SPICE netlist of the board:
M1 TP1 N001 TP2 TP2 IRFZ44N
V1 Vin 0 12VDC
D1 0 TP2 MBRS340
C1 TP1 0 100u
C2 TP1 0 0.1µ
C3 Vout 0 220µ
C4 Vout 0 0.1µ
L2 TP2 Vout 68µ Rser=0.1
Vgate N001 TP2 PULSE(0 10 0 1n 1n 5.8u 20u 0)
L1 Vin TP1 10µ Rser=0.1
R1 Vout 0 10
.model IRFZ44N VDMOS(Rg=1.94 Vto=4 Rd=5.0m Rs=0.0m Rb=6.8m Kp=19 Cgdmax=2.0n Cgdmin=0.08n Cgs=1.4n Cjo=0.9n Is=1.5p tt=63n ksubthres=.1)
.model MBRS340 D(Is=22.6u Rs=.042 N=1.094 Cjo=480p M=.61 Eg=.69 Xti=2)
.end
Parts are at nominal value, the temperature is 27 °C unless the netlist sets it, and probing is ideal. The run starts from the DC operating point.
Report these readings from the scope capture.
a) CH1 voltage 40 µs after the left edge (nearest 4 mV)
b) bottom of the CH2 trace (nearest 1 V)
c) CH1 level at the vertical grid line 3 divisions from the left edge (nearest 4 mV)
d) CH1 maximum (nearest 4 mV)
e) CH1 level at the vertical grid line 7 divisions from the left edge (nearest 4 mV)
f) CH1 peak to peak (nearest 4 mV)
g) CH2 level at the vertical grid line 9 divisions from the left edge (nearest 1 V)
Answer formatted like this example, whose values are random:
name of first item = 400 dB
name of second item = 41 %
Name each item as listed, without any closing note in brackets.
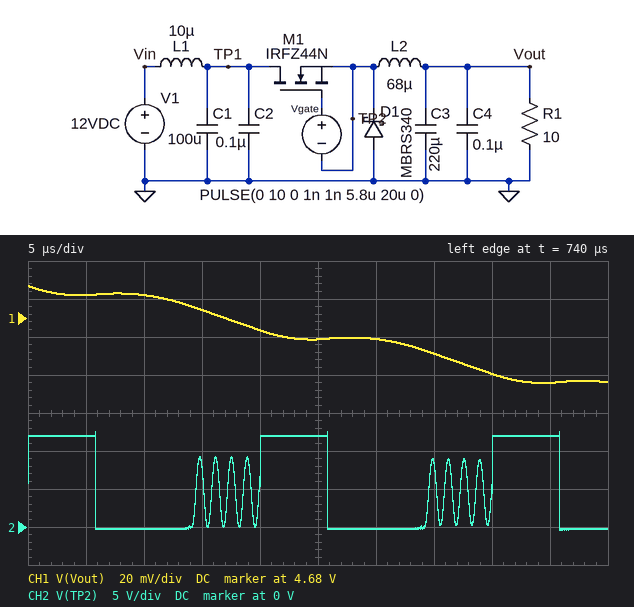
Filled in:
CH1 voltage 40 µs after the left edge = 4.652 V
bottom of the CH2 trace = 0 V
CH1 level at the vertical grid line 3 divisions from the left edge = 4.684 V
CH1 maximum = 4.696 V
CH1 level at the vertical grid line 7 divisions from the left edge = 4.660 V
CH1 peak to peak = 52 mV
CH2 level at the vertical grid line 9 divisions from the left edge = 12 V
